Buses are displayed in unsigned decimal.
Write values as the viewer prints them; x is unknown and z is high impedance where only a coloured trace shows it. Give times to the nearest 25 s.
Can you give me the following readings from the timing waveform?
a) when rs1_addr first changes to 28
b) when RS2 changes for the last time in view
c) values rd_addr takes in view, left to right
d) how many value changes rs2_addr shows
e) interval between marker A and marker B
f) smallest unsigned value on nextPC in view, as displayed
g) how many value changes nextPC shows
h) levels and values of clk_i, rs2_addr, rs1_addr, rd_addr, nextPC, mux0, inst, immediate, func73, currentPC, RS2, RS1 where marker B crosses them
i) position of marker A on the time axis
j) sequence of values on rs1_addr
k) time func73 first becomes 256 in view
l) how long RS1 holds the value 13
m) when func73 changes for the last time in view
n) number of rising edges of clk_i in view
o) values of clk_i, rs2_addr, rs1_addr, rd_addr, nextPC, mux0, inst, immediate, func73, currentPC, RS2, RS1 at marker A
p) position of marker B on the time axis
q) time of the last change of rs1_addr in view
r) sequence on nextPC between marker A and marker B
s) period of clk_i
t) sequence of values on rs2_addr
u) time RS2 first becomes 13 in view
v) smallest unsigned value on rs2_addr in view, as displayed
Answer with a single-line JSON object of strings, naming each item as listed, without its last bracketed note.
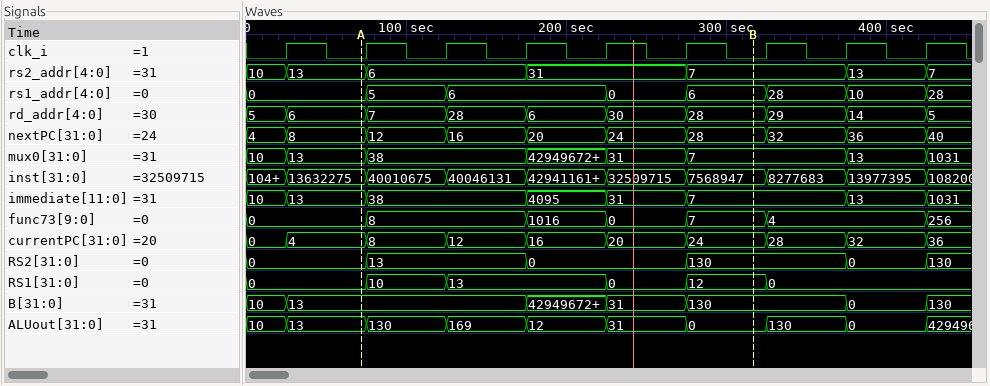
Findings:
{"when rs1_addr first changes to 28": "325 s", "when RS2 changes for the last time in view": "425 s", "values rd_addr takes in view, left to right": "5, 6, 7, 28, 6, 30, 28, 29, 14, 5", "how many value changes rs2_addr shows": "6", "interval between marker A and marker B": "250 s", "smallest unsigned value on nextPC in view, as displayed": "4", "how many value changes nextPC shows": "9", "levels and values of clk_i, rs2_addr, rs1_addr, rd_addr, nextPC, mux0, inst, immediate, func73, currentPC, RS2, RS1 where marker B crosses them": "clk_i=0, rs2_addr=7, rs1_addr=6, rd_addr=28, nextPC=28, mux0=7, inst=7568947, immediate=7, func73=7, currentPC=24, RS2=130, RS1=12", "position of marker A on the time axis": "75 s", "sequence of values on rs1_addr": "0, 5, 6, 0, 6, 28, 10, 28", "time func73 first becomes 256 in view": "425 s", "how long RS1 holds the value 13": "100 s", "when func73 changes for the last time in view": "425 s", "number of rising edges of clk_i in view": "9", "values of clk_i, rs2_addr, rs1_addr, rd_addr, nextPC, mux0, inst, immediate, func73, currentPC, RS2, RS1 at marker A": "clk_i=0, rs2_addr=13, rs1_addr=0, rd_addr=6, nextPC=8, mux0=13, inst=13632275, immediate=13, func73=0, currentPC=4, RS2=0, RS1=0", "position of marker B on the time axis": "325 s", "time of the last change of rs1_addr in view": "425 s", "sequence on nextPC between marker A and marker B": "8, 12, 16, 20, 24, 28", "period of clk_i": "50 s", "sequence of values on rs2_addr": "10, 13, 6, 31, 7, 13, 7", "time RS2 first becomes 13 in view": "75 s", "smallest unsigned value on rs2_addr in view, as displayed": "6"}
